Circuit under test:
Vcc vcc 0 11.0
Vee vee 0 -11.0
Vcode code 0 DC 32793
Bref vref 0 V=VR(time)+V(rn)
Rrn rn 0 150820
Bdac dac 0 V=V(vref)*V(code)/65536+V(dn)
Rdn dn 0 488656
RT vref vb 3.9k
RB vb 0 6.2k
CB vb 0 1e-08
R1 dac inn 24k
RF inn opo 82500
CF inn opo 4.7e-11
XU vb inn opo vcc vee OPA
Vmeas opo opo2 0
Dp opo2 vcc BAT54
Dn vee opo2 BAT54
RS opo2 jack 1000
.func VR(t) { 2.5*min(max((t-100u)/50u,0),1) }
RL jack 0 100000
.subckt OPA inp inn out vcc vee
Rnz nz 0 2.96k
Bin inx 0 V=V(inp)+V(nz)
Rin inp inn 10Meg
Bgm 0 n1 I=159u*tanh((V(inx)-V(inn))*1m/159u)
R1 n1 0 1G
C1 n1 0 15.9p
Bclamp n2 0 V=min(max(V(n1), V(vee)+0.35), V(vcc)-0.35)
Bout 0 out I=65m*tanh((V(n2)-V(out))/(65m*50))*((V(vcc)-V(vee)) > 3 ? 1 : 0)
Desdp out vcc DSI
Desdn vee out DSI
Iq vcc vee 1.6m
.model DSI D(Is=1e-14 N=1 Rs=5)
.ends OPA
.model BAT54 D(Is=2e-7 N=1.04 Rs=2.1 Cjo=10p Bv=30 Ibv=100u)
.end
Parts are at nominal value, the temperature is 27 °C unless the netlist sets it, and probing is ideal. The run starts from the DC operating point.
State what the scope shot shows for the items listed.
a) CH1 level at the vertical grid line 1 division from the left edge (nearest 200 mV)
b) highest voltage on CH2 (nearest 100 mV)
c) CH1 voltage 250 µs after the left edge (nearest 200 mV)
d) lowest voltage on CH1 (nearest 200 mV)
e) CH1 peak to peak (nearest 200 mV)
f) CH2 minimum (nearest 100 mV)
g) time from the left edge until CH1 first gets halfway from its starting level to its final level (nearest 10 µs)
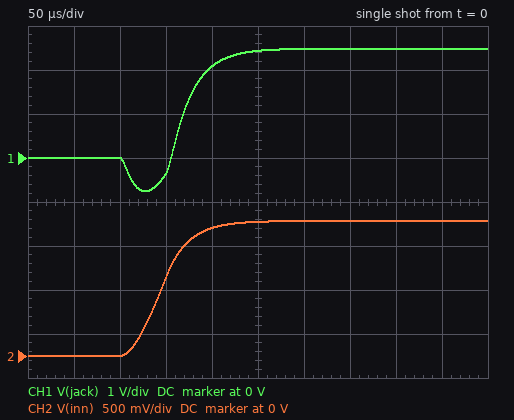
0 V
1.5 V
2.4 V
-800 mV
3.2 V
0 V
170 µs
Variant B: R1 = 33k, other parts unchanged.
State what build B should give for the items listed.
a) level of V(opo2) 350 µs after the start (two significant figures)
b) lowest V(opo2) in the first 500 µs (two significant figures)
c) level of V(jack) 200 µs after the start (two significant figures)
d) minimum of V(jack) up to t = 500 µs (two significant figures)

2.2 V
-480 mV
1.9 V
-470 mV
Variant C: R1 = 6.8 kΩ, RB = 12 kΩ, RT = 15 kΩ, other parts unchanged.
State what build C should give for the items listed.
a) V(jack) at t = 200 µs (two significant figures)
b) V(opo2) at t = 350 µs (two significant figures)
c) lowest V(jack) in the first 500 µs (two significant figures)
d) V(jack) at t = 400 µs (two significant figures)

-5.7 V
-1.1 V
-10 V
-830 mV
